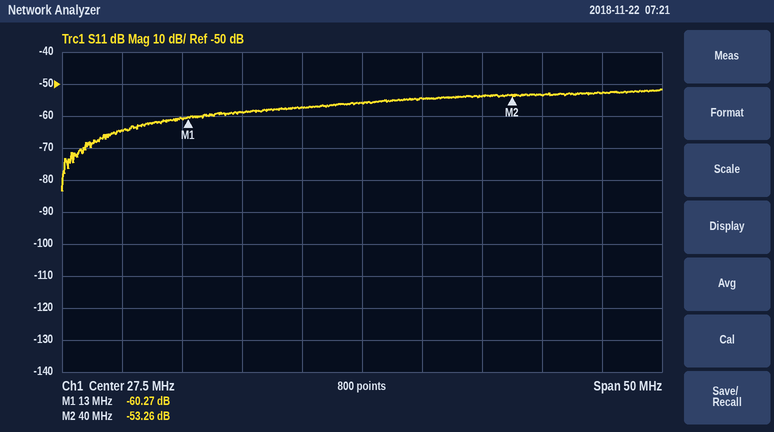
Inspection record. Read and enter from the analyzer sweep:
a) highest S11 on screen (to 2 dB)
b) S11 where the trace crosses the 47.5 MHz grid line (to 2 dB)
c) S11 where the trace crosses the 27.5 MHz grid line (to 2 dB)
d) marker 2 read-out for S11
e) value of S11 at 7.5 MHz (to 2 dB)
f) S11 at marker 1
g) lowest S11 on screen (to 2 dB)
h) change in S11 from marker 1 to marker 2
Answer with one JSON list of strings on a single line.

["-52 dB", "-52 dB", "-56 dB", "-53.26 dB", "-64 dB", "-60.27 dB", "-84 dB", "7.01 dB"]
